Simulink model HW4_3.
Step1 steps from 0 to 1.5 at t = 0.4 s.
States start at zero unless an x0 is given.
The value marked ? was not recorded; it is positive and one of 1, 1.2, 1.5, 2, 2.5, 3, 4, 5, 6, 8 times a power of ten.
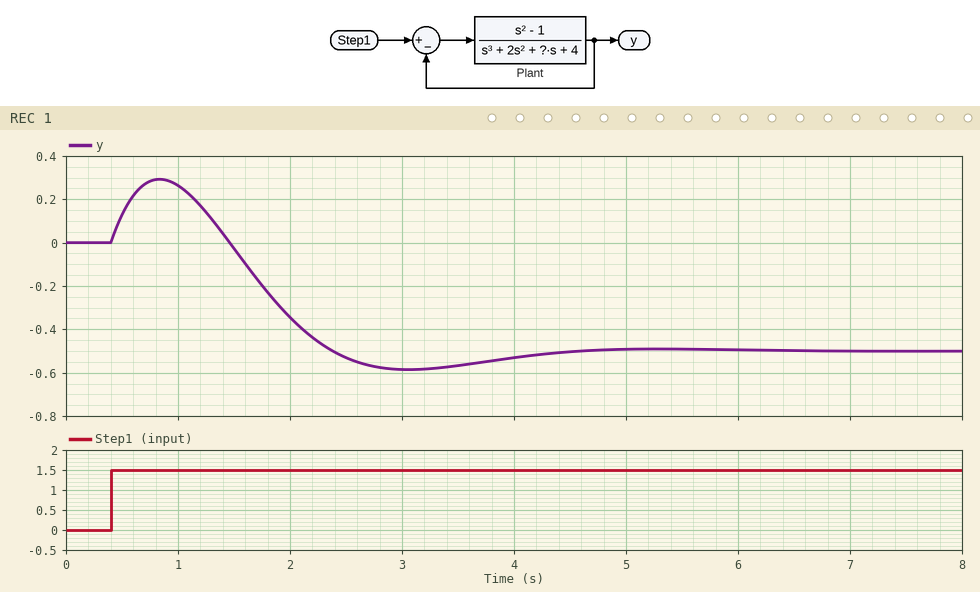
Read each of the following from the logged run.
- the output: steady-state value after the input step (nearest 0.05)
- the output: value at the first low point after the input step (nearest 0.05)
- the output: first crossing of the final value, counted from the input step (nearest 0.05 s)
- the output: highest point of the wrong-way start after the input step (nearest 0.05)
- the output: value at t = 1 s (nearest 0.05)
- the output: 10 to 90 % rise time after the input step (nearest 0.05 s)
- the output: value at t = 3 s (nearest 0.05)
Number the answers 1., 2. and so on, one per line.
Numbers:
1. -0.50
2. -0.60
3. 2.00 s
4. 0.30
5. 0.25
6. 0.70 s
7. -0.60
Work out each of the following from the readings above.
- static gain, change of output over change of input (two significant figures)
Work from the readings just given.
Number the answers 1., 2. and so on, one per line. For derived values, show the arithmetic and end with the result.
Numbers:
1. (-0.5 - 0) / (1.5 - 0) = -0.33
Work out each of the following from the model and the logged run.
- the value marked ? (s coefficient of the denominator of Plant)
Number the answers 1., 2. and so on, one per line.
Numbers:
1. 5
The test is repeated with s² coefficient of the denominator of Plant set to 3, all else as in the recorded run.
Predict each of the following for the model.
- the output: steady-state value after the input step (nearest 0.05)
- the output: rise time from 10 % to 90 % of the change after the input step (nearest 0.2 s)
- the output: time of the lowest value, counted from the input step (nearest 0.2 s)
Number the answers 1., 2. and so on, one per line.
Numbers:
1. -0.50
2. 1.0 s
3. 3.4 s
